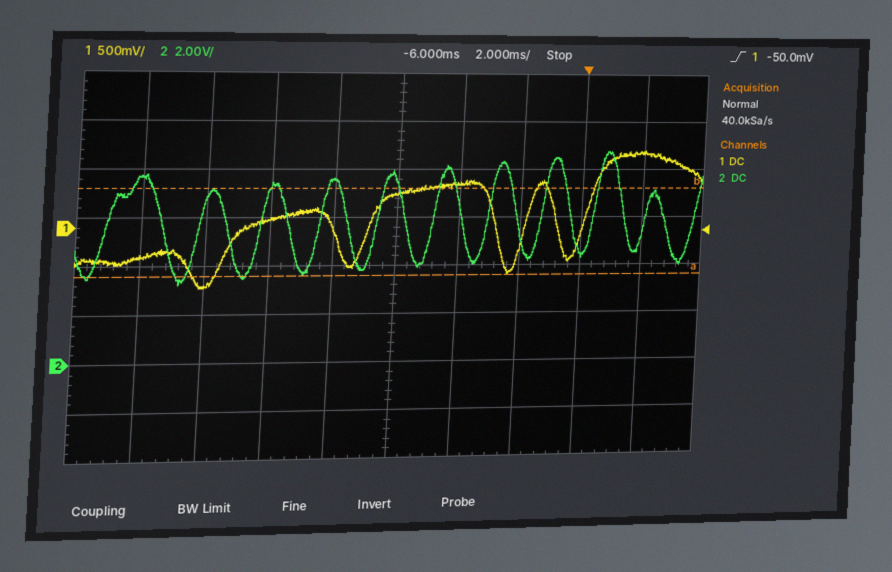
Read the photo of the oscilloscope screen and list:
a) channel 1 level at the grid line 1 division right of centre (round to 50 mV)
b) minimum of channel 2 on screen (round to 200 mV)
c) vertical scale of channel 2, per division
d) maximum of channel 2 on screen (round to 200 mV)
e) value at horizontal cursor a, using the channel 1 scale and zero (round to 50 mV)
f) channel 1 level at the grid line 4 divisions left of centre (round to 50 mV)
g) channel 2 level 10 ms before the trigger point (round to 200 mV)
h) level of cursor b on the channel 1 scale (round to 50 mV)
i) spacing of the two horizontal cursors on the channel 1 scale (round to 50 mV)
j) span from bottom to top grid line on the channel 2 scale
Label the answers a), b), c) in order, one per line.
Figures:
a) 450 mV
b) 3.2 V
c) 2 V
d) 8.8 V
e) -500 mV
f) -300 mV
g) 7.2 V
h) 400 mV
i) 900 mV
j) 16 V
